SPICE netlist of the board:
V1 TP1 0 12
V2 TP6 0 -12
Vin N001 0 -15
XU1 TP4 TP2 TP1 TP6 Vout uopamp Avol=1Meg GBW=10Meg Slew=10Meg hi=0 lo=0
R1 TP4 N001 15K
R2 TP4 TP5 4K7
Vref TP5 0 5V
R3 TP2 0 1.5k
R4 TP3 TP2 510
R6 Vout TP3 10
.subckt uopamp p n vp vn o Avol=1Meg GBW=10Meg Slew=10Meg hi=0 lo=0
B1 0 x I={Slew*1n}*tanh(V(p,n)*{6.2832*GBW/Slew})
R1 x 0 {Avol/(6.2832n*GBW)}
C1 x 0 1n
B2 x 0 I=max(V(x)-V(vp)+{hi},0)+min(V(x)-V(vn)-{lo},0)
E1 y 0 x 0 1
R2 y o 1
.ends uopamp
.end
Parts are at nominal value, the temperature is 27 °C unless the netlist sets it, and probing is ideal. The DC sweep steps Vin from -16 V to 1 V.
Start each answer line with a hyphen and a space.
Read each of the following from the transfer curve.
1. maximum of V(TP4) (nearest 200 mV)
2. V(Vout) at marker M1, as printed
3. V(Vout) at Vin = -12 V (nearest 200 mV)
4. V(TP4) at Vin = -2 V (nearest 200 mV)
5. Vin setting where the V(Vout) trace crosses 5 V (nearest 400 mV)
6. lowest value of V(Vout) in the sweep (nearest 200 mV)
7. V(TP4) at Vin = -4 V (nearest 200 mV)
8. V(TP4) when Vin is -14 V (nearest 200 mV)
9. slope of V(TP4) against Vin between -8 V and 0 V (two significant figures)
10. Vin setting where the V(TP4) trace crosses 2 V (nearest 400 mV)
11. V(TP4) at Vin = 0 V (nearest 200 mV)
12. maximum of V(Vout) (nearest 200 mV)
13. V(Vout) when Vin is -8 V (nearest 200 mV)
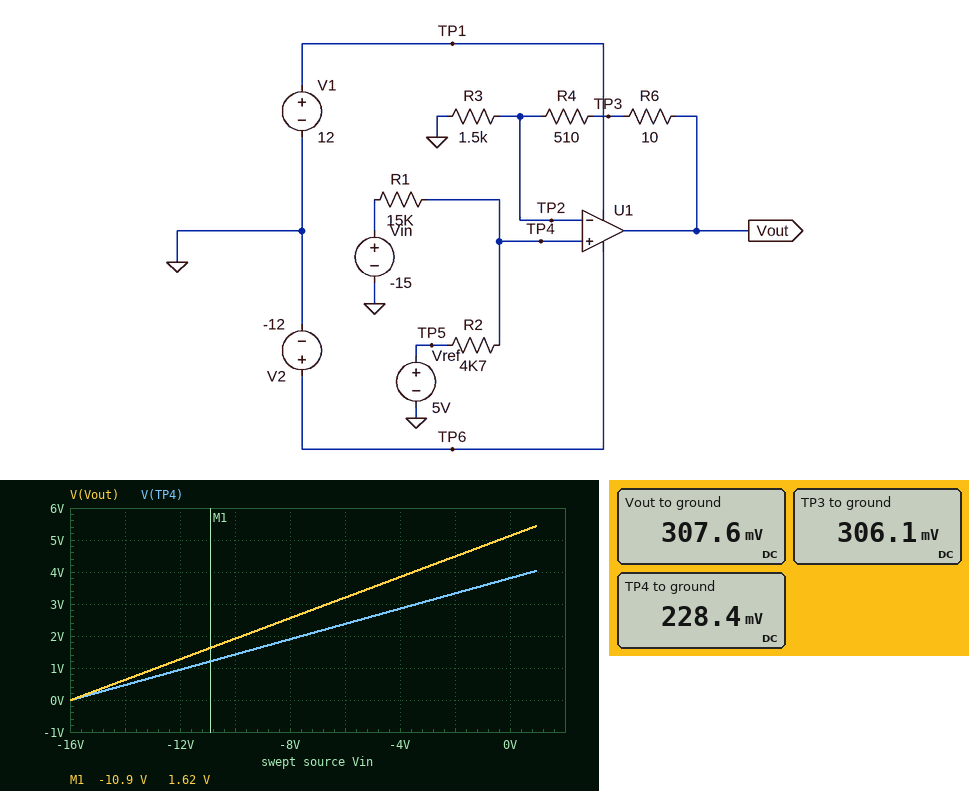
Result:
- 4.0 V
- 1.62 V
- 1.2 V
- 3.4 V
- -400 mV
- 0 V
- 2.8 V
- 400 mV
- 0.24 V/V
- -7.6 V
- 3.8 V
- 5.4 V
- 2.6 V
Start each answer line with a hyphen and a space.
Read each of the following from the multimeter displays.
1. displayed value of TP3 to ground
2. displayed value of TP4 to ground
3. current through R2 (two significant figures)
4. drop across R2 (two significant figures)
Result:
- 306.1 mV
- 228.4 mV
- 1.0 mA
- 4.8 V
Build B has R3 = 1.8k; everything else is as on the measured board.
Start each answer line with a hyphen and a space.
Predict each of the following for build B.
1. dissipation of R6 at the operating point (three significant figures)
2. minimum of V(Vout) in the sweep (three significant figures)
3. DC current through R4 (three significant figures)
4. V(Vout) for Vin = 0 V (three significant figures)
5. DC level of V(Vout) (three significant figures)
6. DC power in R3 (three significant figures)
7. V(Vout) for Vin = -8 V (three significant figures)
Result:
- 161 nW
- -13.1 mV
- 127 µA
- 4.91 V
- 294 mV
- 29.0 µW
- 2.45 V
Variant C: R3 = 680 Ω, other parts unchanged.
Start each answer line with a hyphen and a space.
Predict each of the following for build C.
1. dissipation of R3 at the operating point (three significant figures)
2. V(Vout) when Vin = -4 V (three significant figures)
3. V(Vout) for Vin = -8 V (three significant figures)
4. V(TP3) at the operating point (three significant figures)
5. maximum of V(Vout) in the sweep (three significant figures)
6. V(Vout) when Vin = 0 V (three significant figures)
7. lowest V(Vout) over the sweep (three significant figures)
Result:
- 76.7 µW
- 5.03 V
- 3.35 V
- 400 mV
- 7.14 V
- 6.72 V
- -17.9 mV
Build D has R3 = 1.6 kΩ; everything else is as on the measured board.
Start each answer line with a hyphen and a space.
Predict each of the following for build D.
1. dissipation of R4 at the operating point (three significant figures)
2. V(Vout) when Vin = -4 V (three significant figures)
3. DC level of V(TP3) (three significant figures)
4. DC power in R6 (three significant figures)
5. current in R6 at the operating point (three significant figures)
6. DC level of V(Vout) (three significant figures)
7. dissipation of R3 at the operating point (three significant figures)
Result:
- 10.4 µW
- 3.78 V
- 301 mV
- 204 nW
- 143 µA
- 303 mV
- 32.6 µW
